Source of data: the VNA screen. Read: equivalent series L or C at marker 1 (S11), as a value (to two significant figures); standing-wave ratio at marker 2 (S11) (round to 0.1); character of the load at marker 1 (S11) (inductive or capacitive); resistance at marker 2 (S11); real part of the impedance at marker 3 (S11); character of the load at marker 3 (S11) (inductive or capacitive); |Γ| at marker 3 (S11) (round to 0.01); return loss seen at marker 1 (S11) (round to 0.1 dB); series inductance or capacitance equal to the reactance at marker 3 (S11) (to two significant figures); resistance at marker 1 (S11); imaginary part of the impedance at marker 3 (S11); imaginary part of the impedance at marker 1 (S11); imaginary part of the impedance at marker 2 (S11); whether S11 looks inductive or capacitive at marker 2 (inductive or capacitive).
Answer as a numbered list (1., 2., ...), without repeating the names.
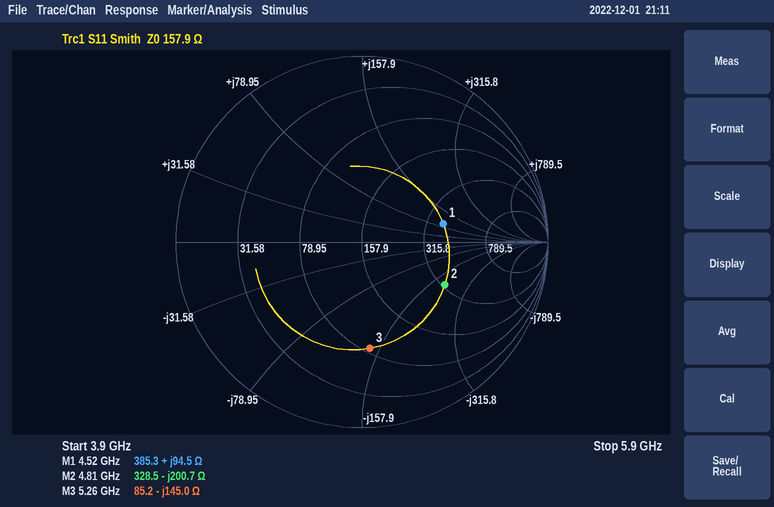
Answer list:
1. 3.3 nH
2. 3.0
3. inductive
4. 328.5 Ω
5. 85.2 Ω
6. capacitive
7. 0.57
8. 7.0 dB
9. 210 fF
10. 385.3 Ω
11. -145.0 Ω
12. +94.5 Ω
13. -200.7 Ω
14. capacitive
